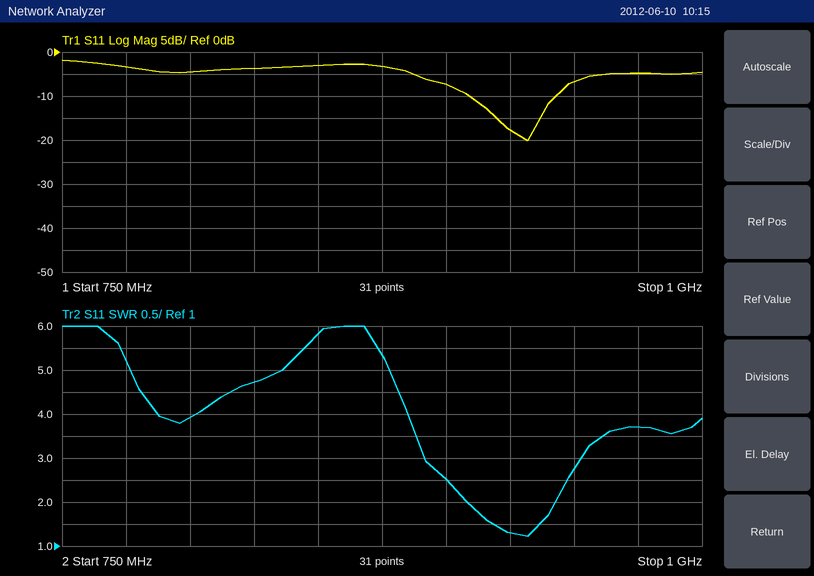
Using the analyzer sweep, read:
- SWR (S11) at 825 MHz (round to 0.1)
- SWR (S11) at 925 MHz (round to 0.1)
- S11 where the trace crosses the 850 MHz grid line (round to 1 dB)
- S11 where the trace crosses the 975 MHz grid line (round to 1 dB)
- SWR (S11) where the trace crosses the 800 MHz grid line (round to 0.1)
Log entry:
4.7
1.3
-3 dB
-5 dB
3.9
